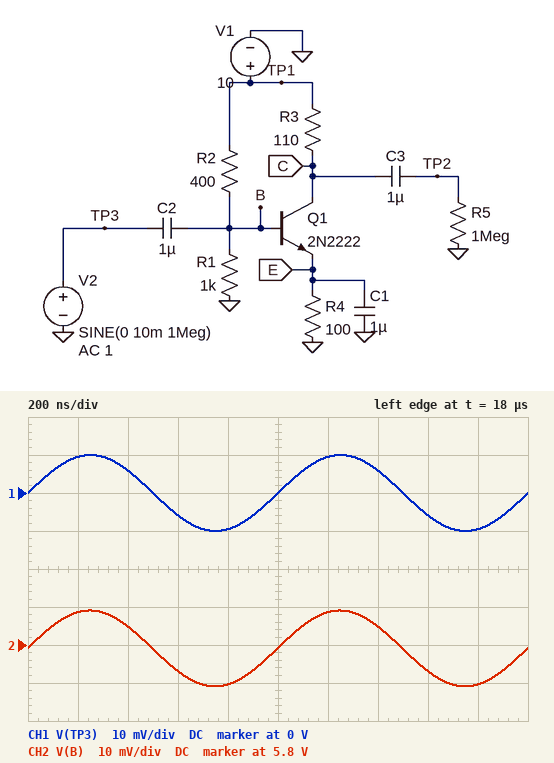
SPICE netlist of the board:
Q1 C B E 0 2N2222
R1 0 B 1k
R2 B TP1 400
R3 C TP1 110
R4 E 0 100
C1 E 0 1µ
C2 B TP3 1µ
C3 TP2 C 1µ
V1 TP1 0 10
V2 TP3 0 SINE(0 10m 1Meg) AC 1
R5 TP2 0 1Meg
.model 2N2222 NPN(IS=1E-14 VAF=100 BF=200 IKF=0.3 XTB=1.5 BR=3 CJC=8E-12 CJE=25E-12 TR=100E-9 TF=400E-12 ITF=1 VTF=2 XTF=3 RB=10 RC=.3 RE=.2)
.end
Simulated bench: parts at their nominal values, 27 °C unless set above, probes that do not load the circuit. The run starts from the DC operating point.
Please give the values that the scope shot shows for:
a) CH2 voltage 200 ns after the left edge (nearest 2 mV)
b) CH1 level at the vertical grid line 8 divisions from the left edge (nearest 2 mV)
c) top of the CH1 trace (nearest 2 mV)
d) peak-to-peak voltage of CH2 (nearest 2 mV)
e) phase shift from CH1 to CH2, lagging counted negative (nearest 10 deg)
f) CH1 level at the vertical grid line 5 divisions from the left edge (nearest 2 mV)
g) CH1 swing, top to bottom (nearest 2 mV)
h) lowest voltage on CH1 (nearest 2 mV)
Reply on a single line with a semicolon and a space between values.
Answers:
5.808 V; -6 mV; 10 mV; 20 mV; 0 deg; 0 V; 20 mV; -10 mV
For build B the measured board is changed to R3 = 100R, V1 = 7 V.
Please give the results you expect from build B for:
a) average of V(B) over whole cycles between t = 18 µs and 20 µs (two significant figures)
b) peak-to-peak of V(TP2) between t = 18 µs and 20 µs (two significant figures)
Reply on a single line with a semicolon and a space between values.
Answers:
4.4 V; 8.2 mV
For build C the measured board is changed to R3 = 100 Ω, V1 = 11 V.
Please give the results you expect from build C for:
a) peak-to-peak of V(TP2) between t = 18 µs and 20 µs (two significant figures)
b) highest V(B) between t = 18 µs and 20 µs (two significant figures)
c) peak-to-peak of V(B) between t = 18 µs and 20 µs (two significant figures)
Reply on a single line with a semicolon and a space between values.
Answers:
3.5 mV; 6.5 V; 20 mV
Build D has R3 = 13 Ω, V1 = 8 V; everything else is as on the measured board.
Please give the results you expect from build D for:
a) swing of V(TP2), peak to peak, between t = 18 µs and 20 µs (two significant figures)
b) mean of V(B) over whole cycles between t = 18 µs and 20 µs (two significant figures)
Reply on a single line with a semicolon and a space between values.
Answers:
290 mV; 5.6 V
